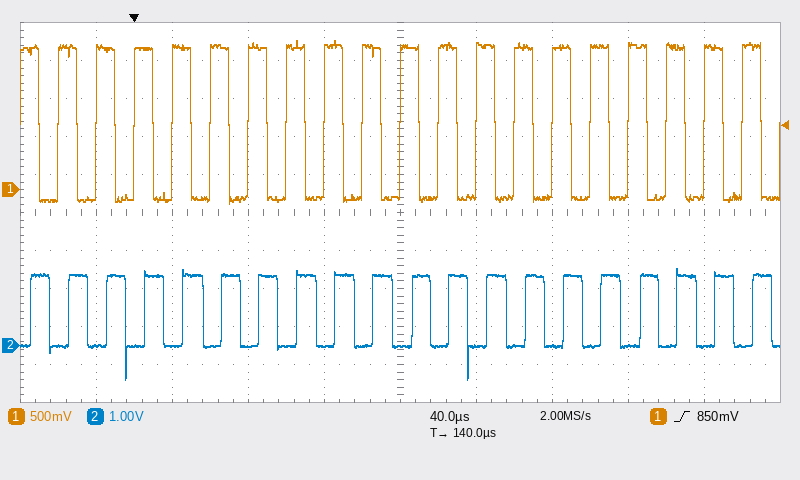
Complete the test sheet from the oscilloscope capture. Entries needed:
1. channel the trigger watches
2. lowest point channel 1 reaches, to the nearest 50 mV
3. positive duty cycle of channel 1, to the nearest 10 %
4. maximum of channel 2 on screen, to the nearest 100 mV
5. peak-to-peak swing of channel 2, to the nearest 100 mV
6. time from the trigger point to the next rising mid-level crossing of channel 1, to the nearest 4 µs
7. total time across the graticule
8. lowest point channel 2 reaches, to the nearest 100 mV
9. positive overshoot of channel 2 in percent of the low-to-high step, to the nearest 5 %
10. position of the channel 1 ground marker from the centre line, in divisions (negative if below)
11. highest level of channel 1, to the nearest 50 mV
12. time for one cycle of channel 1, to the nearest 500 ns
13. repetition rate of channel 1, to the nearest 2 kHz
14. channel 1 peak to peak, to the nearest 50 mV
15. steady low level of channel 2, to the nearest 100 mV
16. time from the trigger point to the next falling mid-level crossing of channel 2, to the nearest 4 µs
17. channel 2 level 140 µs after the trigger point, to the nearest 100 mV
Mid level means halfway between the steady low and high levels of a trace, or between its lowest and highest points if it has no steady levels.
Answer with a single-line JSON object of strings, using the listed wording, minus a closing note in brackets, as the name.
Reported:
{"channel the trigger watches": "channel 1", "lowest point channel 1 reaches, to the nearest 50 mV": "-200 mV", "positive duty cycle of channel 1, to the nearest 10 %": "50 %", "maximum of channel 2 on screen, to the nearest 100 mV": "2.0 V", "peak-to-peak swing of channel 2, to the nearest 100 mV": "2.9 V", "time from the trigger point to the next rising mid-level crossing of channel 1, to the nearest 4 µs": "20 µs", "total time across the graticule": "400 µs", "lowest point channel 2 reaches, to the nearest 100 mV": "-900 mV", "positive overshoot of channel 2 in percent of the low-to-high step, to the nearest 5 %": "10 %", "position of the channel 1 ground marker from the centre line, in divisions": "+0.6 div", "highest level of channel 1, to the nearest 50 mV": "1.95 V", "time for one cycle of channel 1, to the nearest 500 ns": "20.0 µs", "repetition rate of channel 1, to the nearest 2 kHz": "50 kHz", "channel 1 peak to peak, to the nearest 50 mV": "2.15 V", "steady low level of channel 2, to the nearest 100 mV": "0.0 V", "time from the trigger point to the next falling mid-level crossing of channel 2, to the nearest 4 µs": "16 µs", "channel 2 level 140 µs after the trigger point, to the nearest 100 mV": "0.0 V"}
